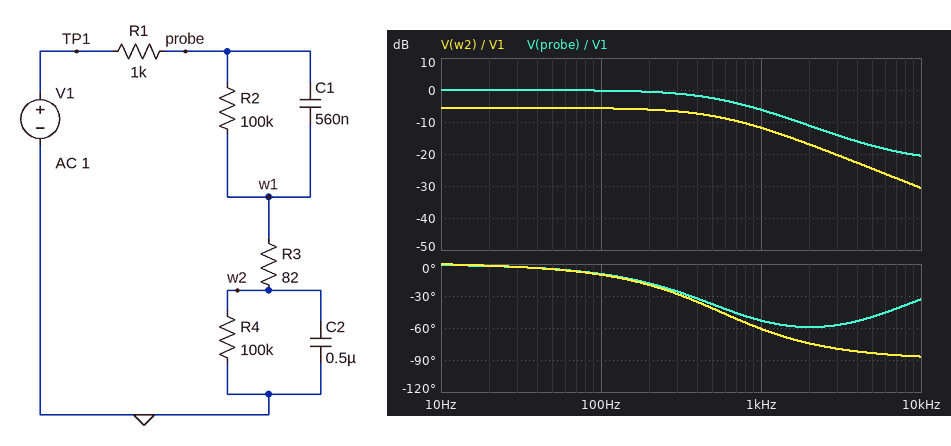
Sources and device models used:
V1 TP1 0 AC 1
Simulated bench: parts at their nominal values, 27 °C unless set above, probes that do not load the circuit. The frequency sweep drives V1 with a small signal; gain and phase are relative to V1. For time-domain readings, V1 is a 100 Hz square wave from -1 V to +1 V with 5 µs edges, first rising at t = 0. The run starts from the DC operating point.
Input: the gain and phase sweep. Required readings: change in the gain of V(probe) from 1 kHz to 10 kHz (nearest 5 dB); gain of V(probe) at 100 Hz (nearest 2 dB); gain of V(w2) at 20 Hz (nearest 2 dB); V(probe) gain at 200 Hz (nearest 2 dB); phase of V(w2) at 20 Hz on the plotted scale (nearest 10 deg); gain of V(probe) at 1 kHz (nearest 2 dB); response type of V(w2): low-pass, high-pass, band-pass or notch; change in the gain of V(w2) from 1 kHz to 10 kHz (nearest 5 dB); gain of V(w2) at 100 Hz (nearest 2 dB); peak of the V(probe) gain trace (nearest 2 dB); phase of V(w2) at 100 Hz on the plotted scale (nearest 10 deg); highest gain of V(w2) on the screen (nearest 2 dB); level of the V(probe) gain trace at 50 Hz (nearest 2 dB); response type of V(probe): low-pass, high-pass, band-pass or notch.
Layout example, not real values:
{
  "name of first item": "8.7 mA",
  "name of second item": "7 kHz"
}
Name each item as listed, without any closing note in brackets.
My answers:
{
  "change in the gain of V(probe) from 1 kHz to 10 kHz": "-15 dB",
  "gain of V(probe) at 100 Hz": "0 dB",
  "gain of V(w2) at 20 Hz": "-6 dB",
  "V(probe) gain at 200 Hz": "0 dB",
  "phase of V(w2) at 20 Hz on the plotted scale": "0 deg",
  "gain of V(probe) at 1 kHz": "-6 dB",
  "response type of V(w2): low-pass, high-pass, band-pass or notch": "low-pass",
  "change in the gain of V(w2) from 1 kHz to 10 kHz": "-20 dB",
  "gain of V(w2) at 100 Hz": "-6 dB",
  "peak of the V(probe) gain trace": "0 dB",
  "phase of V(w2) at 100 Hz on the plotted scale": "-10 deg",
  "highest gain of V(w2) on the screen": "-6 dB",
  "level of the V(probe) gain trace at 50 Hz": "0 dB",
  "response type of V(probe): low-pass, high-pass, band-pass or notch": "low-pass"
}
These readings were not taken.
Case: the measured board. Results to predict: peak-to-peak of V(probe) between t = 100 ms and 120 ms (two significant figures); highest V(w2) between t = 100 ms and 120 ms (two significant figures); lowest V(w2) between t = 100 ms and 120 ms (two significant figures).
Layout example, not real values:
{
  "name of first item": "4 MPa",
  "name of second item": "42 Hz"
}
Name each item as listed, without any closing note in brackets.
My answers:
{
  "peak-to-peak of V(probe) between t = 100 ms and 120 ms": "2.0 V",
  "highest V(w2) between t = 100 ms and 120 ms": "530 mV",
  "lowest V(w2) between t = 100 ms and 120 ms": "-520 mV"
}
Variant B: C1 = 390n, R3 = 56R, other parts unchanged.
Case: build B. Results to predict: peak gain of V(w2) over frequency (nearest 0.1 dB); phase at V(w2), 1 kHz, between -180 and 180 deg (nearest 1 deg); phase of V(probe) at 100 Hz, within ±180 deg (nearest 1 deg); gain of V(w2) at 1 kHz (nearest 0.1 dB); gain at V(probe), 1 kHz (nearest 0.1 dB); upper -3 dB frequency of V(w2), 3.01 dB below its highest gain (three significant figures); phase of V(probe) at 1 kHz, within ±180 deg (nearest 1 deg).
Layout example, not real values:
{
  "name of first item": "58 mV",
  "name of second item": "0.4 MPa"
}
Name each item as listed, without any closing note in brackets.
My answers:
{
  "peak gain of V(w2) over frequency": "-6.1 dB",
  "phase at V(w2), 1 kHz, between -180 and 180 deg": "-55 deg",
  "phase of V(probe) at 100 Hz, within ±180 deg": "-8 deg",
  "gain of V(w2) at 1 kHz": "-12.1 dB",
  "gain at V(probe), 1 kHz": "-4.9 dB",
  "upper -3 dB frequency of V(w2), 3.01 dB below its highest gain": "506 Hz",
  "phase of V(probe) at 1 kHz, within ±180 deg": "-51 deg"
}
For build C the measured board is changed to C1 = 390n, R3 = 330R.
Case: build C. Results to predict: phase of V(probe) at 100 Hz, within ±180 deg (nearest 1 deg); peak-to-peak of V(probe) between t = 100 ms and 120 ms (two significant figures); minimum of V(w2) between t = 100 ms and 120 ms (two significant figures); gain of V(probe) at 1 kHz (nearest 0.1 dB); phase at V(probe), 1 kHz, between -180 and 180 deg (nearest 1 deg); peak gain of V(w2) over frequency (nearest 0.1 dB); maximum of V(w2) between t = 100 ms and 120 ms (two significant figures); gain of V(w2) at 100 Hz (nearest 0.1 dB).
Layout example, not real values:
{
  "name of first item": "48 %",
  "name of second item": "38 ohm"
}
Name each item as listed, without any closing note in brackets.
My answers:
{
  "phase of V(probe) at 100 Hz, within ±180 deg": "-8 deg",
  "peak-to-peak of V(probe) between t = 100 ms and 120 ms": "2.0 V",
  "minimum of V(w2) between t = 100 ms and 120 ms": "-440 mV",
  "gain of V(probe) at 1 kHz": "-5.6 dB",
  "phase at V(probe), 1 kHz, between -180 and 180 deg": "-37 deg",
  "peak gain of V(w2) over frequency": "-6.1 dB",
  "maximum of V(w2) between t = 100 ms and 120 ms": "430 mV",
  "gain of V(w2) at 100 Hz": "-7.4 dB"
}
